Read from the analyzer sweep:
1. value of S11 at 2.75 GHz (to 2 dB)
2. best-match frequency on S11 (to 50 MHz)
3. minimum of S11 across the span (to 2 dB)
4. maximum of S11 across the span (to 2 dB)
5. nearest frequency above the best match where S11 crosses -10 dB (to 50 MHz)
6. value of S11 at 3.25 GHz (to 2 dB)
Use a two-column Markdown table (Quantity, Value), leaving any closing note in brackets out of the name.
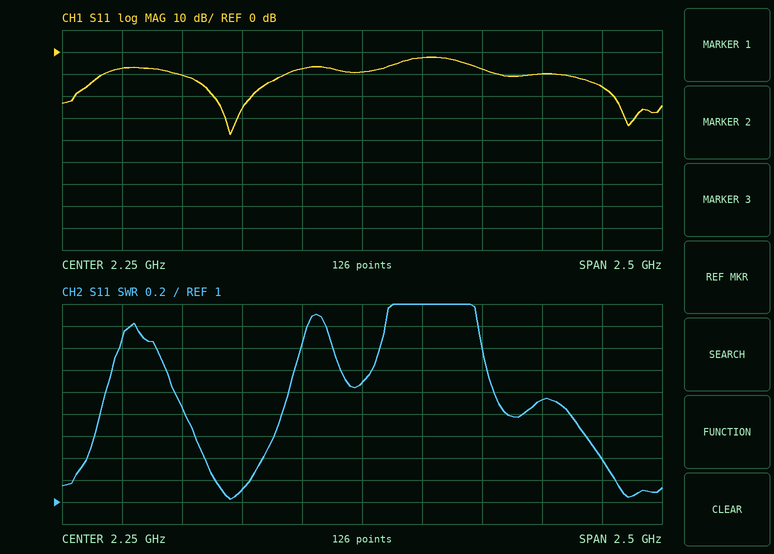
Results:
| Quantity | Value |
|---|---|
| value of S11 at 2.75 GHz | -8 dB |
| best-match frequency on S11 | 1.70 GHz |
| minimum of S11 across the span | -38 dB |
| maximum of S11 across the span | -2 dB |
| nearest frequency above the best match where S11 crosses -10 dB | 1.95 GHz |
| value of S11 at 3.25 GHz | -16 dB |
